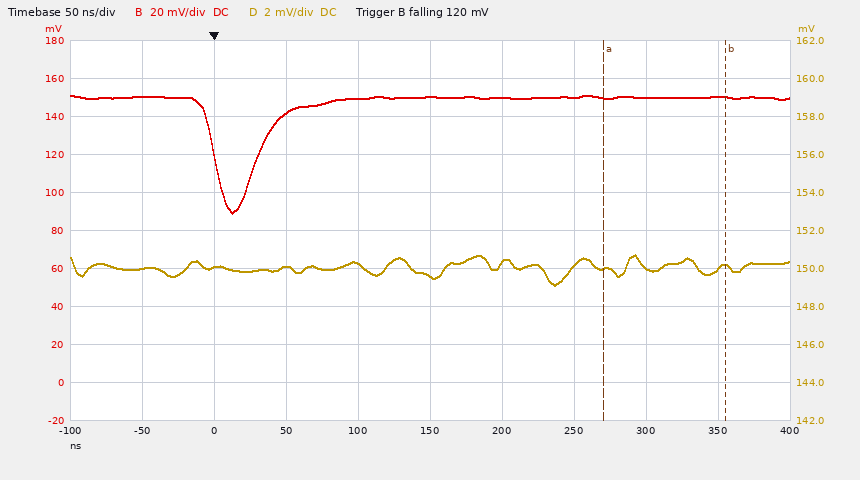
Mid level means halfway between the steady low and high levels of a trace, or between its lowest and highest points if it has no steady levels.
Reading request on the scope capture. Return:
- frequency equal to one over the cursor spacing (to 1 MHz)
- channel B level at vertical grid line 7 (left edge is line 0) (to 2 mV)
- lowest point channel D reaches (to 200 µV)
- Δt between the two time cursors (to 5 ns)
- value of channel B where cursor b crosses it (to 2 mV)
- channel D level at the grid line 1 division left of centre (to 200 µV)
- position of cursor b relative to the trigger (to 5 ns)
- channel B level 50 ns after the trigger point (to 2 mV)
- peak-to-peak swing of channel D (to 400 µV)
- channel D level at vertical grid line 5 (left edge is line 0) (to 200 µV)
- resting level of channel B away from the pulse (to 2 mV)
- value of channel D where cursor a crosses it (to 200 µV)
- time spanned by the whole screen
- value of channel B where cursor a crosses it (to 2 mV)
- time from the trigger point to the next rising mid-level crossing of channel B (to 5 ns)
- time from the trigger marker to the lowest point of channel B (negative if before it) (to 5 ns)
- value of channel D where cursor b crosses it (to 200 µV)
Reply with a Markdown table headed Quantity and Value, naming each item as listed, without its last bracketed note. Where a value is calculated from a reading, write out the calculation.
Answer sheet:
| Quantity | Value |
|---|---|
| frequency equal to one over the cursor spacing | 1 / 85 ns ≈ 12 MHz |
| channel B level at vertical grid line 7 (left edge is line 0) | 150 mV |
| lowest point channel D reaches | 149.2 mV |
| Δt between the two time cursors | 85 ns |
| value of channel B where cursor b crosses it | 150 mV |
| channel D level at the grid line 1 division left of centre | 150.2 mV |
| position of cursor b relative to the trigger | +355 ns |
| channel B level 50 ns after the trigger point | 142 mV |
| peak-to-peak swing of channel D | 1.6 mV |
| channel D level at vertical grid line 5 (left edge is line 0) | 149.6 mV |
| resting level of channel B away from the pulse | 150 mV |
| value of channel D where cursor a crosses it | 150.0 mV |
| time spanned by the whole screen | 500 ns |
| value of channel B where cursor a crosses it | 150 mV |
| time from the trigger point to the next rising mid-level crossing of channel B | 30 ns |
| time from the trigger marker to the lowest point of channel B (negative if before it) | +15 ns |
| value of channel D where cursor b crosses it | 150.2 mV |
